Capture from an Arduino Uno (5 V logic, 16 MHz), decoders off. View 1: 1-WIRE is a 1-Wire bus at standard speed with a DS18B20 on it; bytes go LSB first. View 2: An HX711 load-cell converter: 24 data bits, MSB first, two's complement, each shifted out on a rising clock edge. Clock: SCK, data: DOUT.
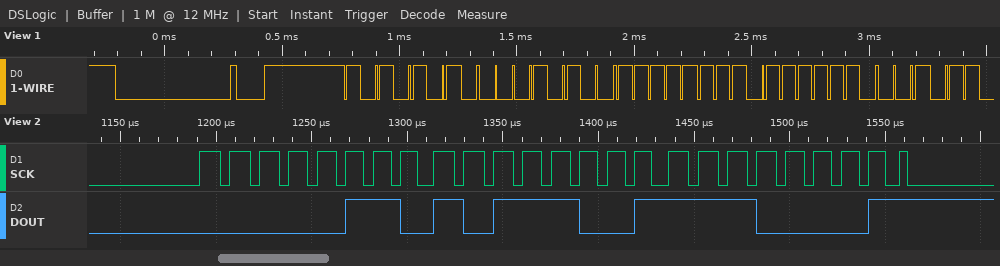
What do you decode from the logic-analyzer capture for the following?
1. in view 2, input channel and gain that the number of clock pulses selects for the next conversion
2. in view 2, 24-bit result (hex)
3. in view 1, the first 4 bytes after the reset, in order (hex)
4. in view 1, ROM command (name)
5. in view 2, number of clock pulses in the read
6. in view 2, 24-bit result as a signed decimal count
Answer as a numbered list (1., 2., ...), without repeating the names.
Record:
1. channel A, gain 128
2. 0x06B9E1
3. 55 28 FF 7E
4. Match ROM
5. 25
6. 440801
